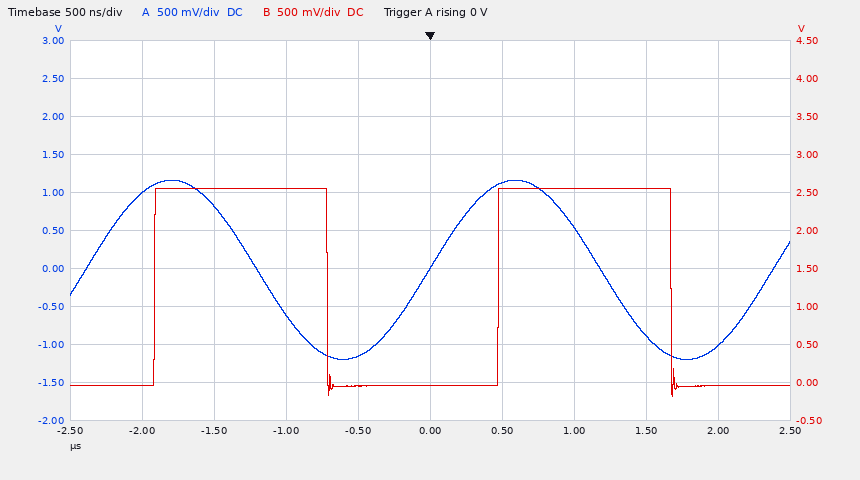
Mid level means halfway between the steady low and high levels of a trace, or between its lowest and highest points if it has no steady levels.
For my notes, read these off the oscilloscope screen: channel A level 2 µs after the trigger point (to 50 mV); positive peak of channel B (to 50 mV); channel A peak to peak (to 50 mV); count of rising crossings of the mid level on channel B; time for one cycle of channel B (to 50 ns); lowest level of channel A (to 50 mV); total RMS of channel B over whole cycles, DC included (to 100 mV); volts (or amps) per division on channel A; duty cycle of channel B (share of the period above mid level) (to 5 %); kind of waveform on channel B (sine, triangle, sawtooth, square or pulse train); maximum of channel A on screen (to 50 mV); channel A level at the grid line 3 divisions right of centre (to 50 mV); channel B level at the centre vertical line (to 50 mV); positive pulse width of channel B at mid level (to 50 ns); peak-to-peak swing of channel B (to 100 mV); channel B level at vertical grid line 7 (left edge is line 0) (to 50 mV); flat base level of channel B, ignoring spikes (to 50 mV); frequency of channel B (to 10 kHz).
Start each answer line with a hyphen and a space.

- -1.00 V
- 2.55 V
- 2.35 V
- 2
- 2.40 µs
- -1.20 V
- 1.8 V
- 500 mV
- 50 %
- square
- 1.15 V
- -900 mV
- -50 mV
- 1.20 µs
- 2.70 V
- 2.55 V
- -50 mV
- 420 kHz
